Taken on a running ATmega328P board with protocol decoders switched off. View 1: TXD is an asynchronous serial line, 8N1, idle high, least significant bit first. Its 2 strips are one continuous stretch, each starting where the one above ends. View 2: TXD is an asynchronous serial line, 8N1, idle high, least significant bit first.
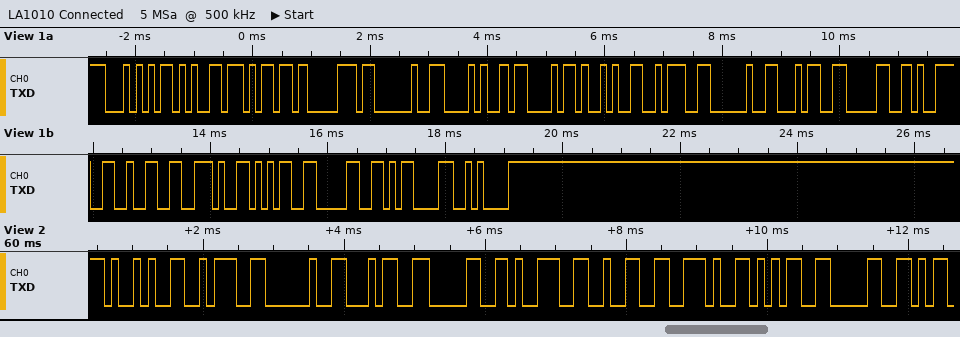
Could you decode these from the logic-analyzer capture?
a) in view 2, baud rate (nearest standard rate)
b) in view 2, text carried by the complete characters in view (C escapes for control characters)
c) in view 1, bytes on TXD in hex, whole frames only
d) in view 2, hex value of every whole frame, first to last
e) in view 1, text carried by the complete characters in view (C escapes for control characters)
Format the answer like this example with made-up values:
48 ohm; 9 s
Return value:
9600 baud; "): 4092.50"; 54 65 6D 70 20 28 43 29 3A 20 34 30 39 32 2E 35 30 0D 0A; 29 3A 20 34 30 39 32 2E 35 30; "Temp (C): 4092.50\r\n"
